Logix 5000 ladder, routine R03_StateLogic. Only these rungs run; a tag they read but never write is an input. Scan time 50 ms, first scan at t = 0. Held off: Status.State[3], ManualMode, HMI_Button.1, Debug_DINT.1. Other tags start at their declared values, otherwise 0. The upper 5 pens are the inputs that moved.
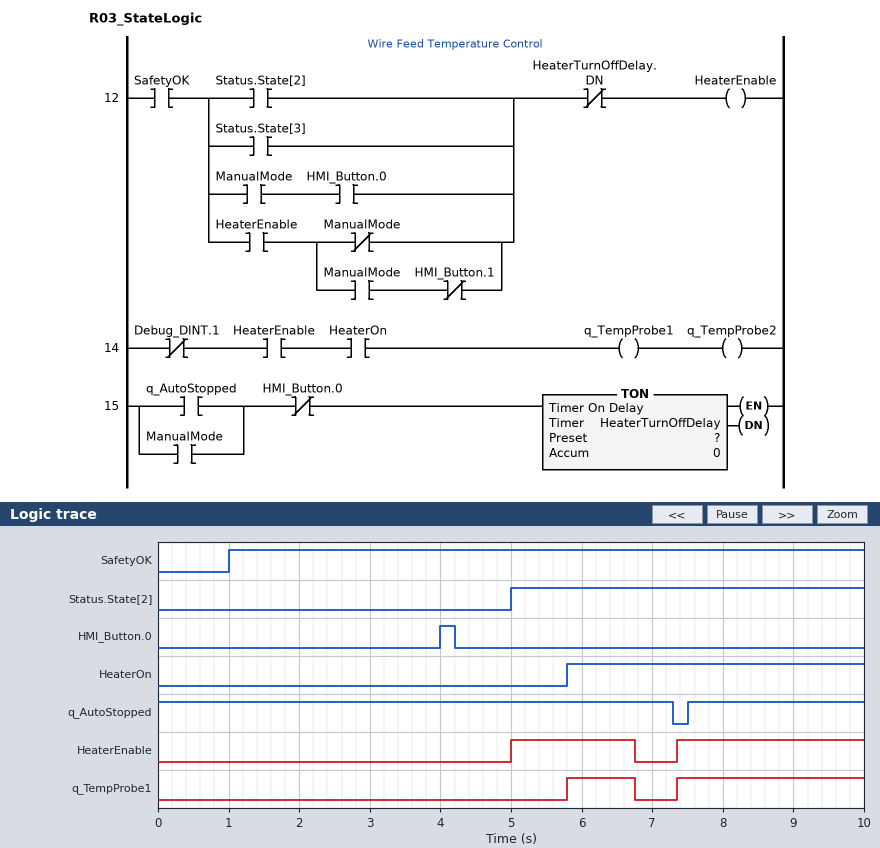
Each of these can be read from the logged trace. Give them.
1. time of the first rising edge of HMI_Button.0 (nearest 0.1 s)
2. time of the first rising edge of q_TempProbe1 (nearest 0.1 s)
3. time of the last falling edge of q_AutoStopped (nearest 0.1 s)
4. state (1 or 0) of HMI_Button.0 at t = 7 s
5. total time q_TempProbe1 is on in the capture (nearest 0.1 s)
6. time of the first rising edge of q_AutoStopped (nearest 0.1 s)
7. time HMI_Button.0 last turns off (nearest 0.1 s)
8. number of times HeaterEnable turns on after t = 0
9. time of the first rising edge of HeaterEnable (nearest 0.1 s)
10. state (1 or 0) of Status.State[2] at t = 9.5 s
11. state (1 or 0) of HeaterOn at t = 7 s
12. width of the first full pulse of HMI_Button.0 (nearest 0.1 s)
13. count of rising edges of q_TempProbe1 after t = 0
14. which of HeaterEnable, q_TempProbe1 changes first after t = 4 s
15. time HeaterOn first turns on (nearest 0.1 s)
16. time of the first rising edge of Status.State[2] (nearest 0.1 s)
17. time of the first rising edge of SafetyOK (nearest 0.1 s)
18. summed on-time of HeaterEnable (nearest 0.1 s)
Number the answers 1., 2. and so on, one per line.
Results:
1. 4.0 s
2. 5.8 s
3. 7.3 s
4. 0
5. 3.6 s
6. 7.5 s
7. 4.2 s
8. 2
9. 5.0 s
10. 1
11. 1
12. 0.2 s
13. 2
14. HeaterEnable
15. 5.8 s
16. 5.0 s
17. 1.0 s
18. 4.4 s
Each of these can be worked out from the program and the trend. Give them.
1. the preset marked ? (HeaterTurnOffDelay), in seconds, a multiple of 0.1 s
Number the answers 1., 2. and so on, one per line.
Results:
1. 2.5 s
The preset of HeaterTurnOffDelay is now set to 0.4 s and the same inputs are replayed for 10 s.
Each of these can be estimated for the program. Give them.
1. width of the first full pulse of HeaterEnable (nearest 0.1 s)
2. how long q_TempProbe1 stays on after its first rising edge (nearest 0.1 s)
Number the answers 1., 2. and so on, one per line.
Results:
1. 0.6 s
2. 0.6 s
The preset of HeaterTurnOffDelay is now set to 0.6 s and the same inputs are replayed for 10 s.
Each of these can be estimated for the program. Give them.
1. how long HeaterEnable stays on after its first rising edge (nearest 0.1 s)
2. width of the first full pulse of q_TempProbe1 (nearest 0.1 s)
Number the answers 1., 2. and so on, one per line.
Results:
1. 0.8 s
2. 0.8 s
